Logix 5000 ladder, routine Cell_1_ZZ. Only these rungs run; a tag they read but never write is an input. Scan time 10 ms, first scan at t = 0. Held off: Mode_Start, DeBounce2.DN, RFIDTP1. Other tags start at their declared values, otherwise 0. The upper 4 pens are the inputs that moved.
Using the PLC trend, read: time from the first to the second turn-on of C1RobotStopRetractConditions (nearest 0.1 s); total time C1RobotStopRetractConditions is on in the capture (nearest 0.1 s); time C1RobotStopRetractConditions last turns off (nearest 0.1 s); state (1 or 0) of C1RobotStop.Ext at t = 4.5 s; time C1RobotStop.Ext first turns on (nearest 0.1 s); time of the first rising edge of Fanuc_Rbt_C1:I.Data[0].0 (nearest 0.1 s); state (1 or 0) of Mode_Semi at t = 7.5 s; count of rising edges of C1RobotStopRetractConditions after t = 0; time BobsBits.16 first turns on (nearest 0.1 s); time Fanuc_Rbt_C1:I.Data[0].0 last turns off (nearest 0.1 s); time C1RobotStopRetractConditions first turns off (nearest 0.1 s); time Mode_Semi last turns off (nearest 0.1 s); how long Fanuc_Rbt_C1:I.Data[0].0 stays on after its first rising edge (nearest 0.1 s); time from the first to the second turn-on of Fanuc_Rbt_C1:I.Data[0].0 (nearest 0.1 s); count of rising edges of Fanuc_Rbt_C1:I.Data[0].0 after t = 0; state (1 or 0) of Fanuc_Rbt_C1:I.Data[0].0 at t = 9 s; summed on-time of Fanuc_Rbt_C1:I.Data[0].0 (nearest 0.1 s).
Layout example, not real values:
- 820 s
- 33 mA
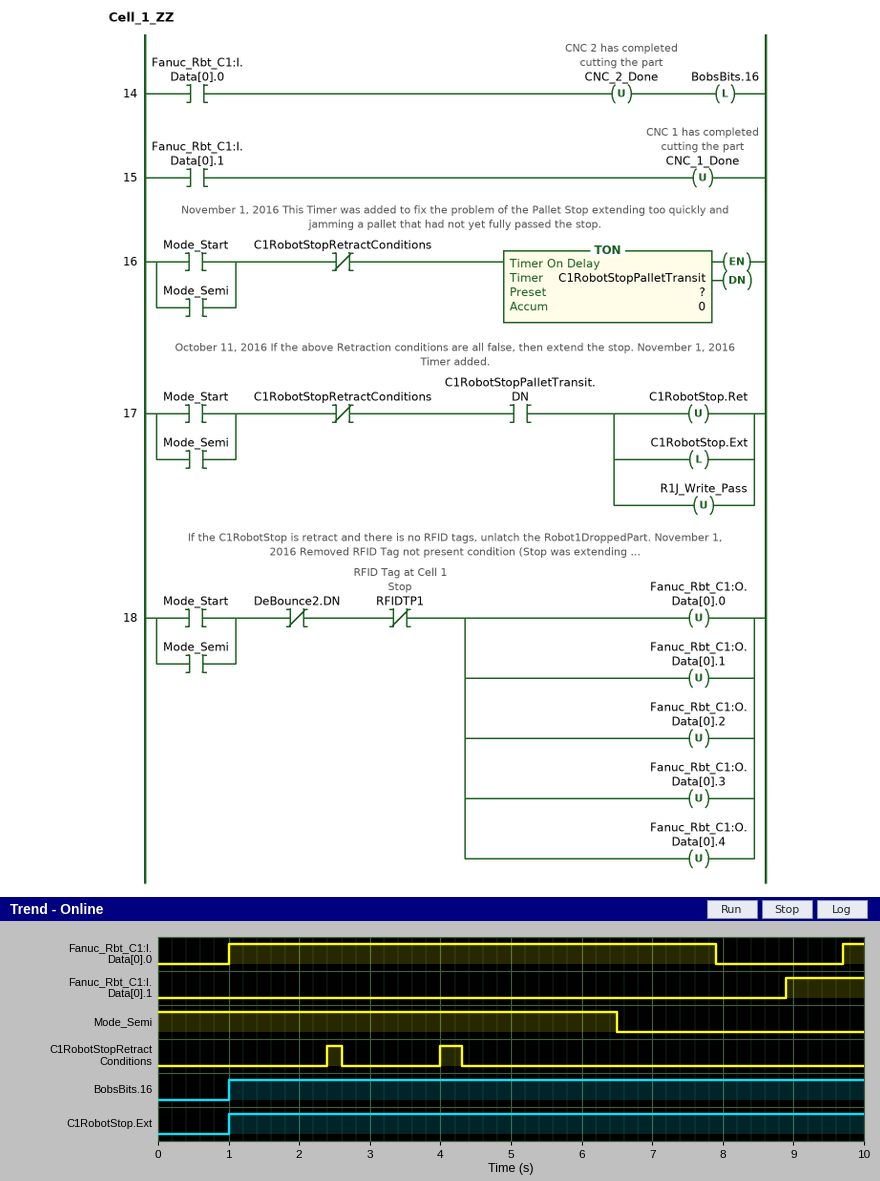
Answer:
- 1.6 s
- 0.5 s
- 4.3 s
- 1
- 1.0 s
- 1.0 s
- 0
- 2
- 1.0 s
- 7.9 s
- 2.6 s
- 6.5 s
- 6.9 s
- 8.7 s
- 2
- 0
- 7.2 s
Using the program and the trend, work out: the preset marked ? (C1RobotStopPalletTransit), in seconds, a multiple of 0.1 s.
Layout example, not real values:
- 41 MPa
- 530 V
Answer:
- 1.0 s
